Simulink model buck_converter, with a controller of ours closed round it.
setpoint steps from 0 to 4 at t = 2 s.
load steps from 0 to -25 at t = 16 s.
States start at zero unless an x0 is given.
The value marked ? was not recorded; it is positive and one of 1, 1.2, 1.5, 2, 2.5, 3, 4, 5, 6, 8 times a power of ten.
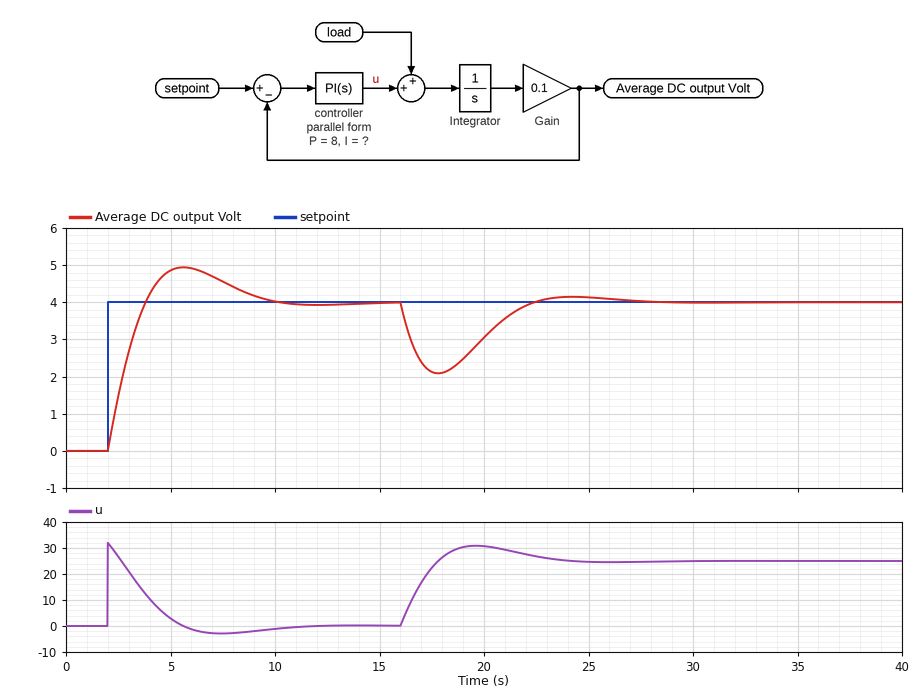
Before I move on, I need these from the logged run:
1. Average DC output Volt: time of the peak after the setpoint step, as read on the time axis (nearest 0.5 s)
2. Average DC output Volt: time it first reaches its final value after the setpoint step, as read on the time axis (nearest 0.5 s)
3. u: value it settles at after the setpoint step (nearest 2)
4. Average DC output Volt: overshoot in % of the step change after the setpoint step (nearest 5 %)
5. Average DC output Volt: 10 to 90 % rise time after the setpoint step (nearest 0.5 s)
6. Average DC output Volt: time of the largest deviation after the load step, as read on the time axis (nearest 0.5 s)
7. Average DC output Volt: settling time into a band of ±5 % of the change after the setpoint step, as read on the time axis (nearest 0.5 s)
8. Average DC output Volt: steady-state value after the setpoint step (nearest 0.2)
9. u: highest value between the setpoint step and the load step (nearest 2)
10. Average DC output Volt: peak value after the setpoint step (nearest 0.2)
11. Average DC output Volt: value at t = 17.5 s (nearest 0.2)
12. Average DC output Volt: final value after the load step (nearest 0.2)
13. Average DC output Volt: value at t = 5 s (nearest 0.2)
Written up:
5.5 s
4.0 s
0
25 %
1.5 s
18.0 s
9.0 s
4.0
32
5.0
2.2
4.0
4.8
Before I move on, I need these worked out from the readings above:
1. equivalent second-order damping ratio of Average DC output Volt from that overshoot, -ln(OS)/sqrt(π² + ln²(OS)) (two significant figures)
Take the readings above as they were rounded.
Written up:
0.40
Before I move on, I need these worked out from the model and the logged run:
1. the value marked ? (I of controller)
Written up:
4
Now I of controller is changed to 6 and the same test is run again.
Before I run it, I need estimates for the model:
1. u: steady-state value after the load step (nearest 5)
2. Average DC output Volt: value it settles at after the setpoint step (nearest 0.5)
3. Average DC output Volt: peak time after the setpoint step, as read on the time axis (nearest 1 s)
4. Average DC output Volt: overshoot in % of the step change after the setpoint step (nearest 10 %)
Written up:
25
4.0
5 s
30 %
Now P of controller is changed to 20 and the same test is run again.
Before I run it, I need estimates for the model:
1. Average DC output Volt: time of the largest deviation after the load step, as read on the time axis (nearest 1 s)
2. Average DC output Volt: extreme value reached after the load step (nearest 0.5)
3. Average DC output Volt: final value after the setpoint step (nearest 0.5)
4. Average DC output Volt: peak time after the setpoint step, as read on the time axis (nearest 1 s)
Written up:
17 s
3.0
4.0
5 s
